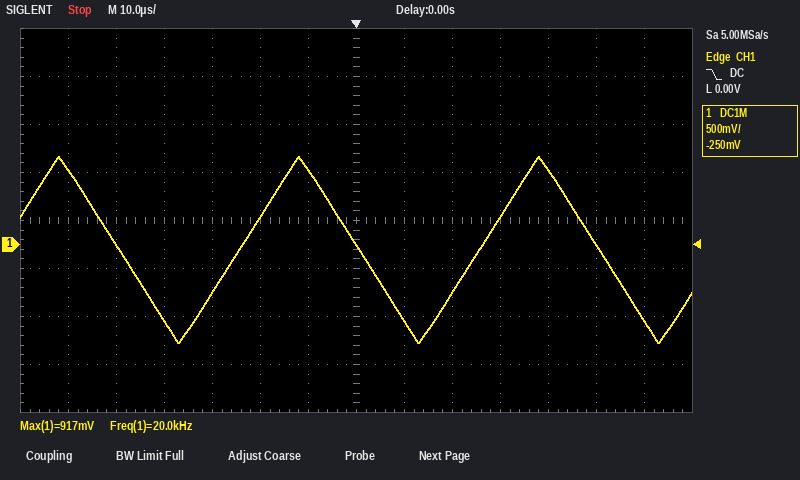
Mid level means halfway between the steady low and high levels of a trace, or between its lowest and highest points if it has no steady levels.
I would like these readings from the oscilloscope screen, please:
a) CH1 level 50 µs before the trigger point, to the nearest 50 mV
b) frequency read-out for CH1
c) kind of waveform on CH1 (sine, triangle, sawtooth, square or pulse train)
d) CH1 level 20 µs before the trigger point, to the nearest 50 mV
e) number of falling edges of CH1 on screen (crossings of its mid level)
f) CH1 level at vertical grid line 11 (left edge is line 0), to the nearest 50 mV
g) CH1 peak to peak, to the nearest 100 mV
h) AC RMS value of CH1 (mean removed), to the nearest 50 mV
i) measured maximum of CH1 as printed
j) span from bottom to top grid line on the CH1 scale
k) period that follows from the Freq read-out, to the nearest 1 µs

0 mV
20.0 kHz
triangle
300 mV
3
800 mV
1.90 V
550 mV
917 mV
4 V
50 µs
